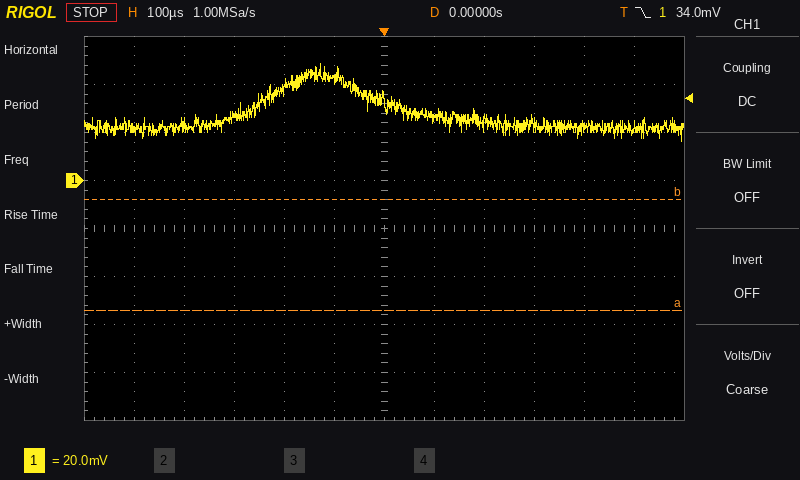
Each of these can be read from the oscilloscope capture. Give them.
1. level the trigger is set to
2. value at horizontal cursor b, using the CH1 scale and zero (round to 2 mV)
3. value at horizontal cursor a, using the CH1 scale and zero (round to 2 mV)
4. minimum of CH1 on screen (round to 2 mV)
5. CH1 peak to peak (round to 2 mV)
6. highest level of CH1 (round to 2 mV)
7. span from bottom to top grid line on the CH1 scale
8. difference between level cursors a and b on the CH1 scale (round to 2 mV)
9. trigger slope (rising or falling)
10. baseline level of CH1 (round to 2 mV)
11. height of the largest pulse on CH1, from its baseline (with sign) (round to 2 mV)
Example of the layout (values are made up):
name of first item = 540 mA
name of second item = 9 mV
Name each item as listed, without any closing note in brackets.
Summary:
level the trigger is set to = 34.0 mV
value at horizontal cursor b, using the CH1 scale and zero = -8 mV
value at horizontal cursor a, using the CH1 scale and zero = -54 mV
minimum of CH1 on screen = 16 mV
CH1 peak to peak = 32 mV
highest level of CH1 = 48 mV
span from bottom to top grid line on the CH1 scale = 160 mV
difference between level cursors a and b on the CH1 scale = 46 mV
trigger slope = falling
baseline level of CH1 = 22 mV
height of the largest pulse on CH1, from its baseline (with sign) = +26 mV
